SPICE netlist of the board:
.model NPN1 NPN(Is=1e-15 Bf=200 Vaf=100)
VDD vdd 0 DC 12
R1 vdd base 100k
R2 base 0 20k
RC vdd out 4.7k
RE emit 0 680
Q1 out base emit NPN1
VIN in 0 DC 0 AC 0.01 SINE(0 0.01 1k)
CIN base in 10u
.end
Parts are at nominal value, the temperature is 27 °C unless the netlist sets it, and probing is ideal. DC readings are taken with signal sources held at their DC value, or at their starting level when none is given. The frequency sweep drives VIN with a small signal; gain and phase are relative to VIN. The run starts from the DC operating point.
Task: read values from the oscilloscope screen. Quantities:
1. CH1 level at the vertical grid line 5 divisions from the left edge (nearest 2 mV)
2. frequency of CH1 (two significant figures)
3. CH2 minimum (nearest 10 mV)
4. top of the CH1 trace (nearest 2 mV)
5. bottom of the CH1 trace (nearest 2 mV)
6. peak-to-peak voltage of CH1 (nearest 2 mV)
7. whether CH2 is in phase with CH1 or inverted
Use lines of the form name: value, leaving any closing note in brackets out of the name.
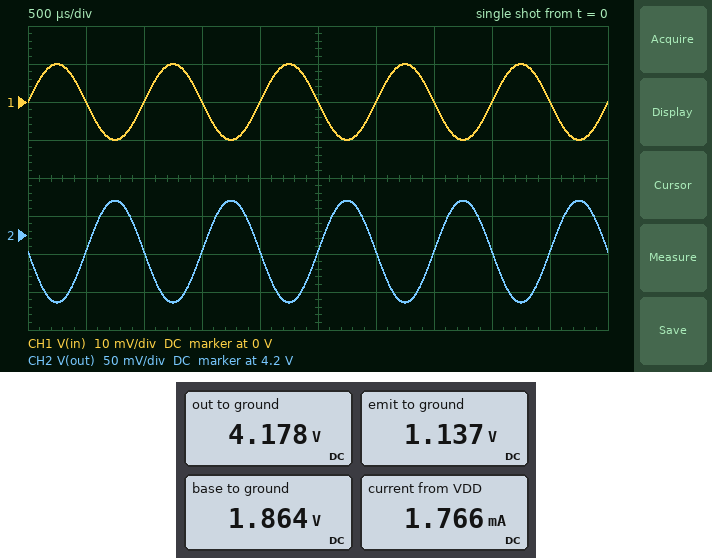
CH1 level at the vertical grid line 5 divisions from the left edge: 0 V
frequency of CH1: 1.0 kHz
CH2 minimum: 4.11 V
top of the CH1 trace: 10 mV
bottom of the CH1 trace: -10 mV
peak-to-peak voltage of CH1: 20 mV
whether CH2 is in phase with CH1 or inverted: inverted
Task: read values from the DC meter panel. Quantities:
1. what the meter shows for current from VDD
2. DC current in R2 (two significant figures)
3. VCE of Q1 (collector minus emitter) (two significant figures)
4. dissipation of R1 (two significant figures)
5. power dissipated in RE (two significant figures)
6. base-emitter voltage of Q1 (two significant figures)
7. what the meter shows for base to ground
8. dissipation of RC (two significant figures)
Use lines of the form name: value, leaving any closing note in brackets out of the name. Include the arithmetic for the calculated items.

what the meter shows for current from VDD: 1.766 mA
DC current in R2: (1.864 V) / 20 kΩ = 93 µA
VCE of Q1 (collector minus emitter): 4.178 V - 1.137 V = 3.0 V
dissipation of R1: (12 V - 1.864 V)^2 / 100 kΩ = 1.0 mW
power dissipated in RE: (1.137 V)^2 / 680 Ω = 1.9 mW
base-emitter voltage of Q1: 1.864 V - 1.137 V = 730 mV
what the meter shows for base to ground: 1.864 V
dissipation of RC: (12 V - 4.178 V)^2 / 4.7 kΩ = 13 mW
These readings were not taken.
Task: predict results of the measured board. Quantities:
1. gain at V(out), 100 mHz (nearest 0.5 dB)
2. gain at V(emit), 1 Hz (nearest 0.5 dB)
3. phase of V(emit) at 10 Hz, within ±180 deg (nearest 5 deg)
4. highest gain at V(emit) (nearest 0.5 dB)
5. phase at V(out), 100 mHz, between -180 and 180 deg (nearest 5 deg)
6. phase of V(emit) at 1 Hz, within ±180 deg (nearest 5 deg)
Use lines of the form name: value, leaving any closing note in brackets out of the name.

gain at V(out), 100 mHz: -4.0 dB
gain at V(emit), 1 Hz: -3.5 dB
phase of V(emit) at 10 Hz, within ±180 deg: 5 deg
highest gain at V(emit): 0 dB
phase at V(out), 100 mHz, between -180 and 180 deg: -95 deg
phase of V(emit) at 1 Hz, within ±180 deg: 45 deg
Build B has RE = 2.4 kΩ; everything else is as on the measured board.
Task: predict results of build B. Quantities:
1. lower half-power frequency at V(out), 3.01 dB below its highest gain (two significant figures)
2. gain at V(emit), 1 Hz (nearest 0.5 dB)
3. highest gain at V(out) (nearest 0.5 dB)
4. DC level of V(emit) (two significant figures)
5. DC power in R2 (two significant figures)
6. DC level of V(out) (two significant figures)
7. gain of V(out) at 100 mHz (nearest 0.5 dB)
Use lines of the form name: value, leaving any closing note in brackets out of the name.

lower half-power frequency at V(out), 3.01 dB below its highest gain: 990 mHz
gain at V(emit), 1 Hz: -3.0 dB
highest gain at V(out): 5.5 dB
DC level of V(emit): 1.3 V
DC power in R2: 190 µW
DC level of V(out): 9.5 V
gain of V(out) at 100 mHz: -14.5 dB
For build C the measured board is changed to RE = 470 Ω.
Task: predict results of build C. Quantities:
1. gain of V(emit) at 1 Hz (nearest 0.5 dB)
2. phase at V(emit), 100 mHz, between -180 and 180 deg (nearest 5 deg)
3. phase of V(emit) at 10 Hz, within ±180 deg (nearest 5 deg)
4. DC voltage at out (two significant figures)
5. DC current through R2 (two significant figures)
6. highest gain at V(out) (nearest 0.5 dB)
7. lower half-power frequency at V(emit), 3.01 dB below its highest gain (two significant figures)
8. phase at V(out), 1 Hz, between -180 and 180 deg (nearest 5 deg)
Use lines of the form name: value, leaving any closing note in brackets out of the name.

gain of V(emit) at 1 Hz: -6.5 dB
phase at V(emit), 100 mHz, between -180 and 180 deg: 85 deg
phase of V(emit) at 10 Hz, within ±180 deg: 10 deg
DC voltage at out: 1.3 V
DC current through R2: 90 µA
highest gain at V(out): 19.5 dB
lower half-power frequency at V(emit), 3.01 dB below its highest gain: 1.8 Hz
phase at V(out), 1 Hz, between -180 and 180 deg: -120 deg
